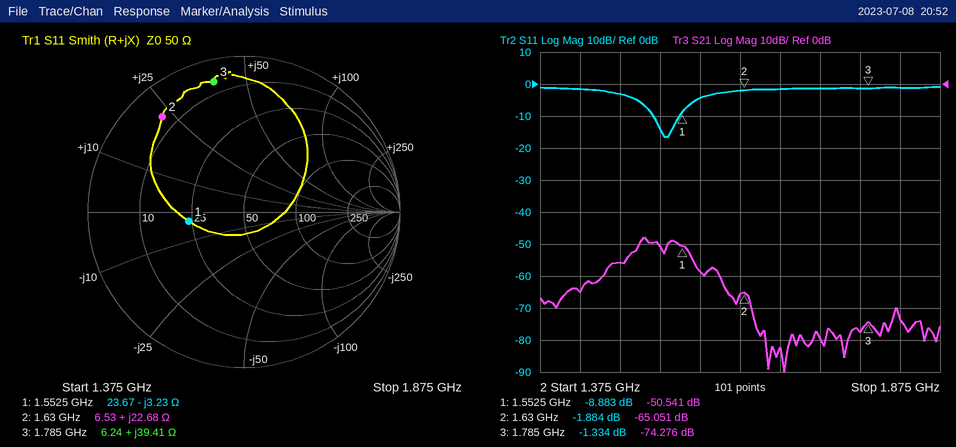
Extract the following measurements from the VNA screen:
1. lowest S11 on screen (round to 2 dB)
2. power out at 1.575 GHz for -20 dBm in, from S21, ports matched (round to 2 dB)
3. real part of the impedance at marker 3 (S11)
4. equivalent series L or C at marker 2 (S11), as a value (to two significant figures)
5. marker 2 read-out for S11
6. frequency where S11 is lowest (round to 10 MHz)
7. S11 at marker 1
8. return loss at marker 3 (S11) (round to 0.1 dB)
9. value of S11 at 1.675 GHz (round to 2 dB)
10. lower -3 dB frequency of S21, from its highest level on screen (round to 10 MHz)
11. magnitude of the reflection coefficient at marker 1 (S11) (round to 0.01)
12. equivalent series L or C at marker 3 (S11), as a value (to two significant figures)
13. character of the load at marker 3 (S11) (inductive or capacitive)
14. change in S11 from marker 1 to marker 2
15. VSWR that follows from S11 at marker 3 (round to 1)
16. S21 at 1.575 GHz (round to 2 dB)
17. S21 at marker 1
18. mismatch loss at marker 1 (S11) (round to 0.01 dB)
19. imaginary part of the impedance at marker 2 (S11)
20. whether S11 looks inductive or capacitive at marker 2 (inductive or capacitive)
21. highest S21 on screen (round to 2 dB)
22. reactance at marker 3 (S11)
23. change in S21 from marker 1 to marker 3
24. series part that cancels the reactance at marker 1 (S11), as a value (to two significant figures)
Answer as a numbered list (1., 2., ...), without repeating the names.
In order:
1. -16 dB
2. -78 dBm
3. 6.24 Ω
4. 2.2 nH
5. -1.884 dB
6. 1.53 GHz
7. -8.883 dB
8. 1.3 dB
9. -2 dB
10. 1.50 GHz
11. 0.36
12. 3.5 nH
13. inductive
14. 6.999 dB
15. 13
16. -58 dB
17. -50.541 dB
18. 0.60 dB
19. +22.68 Ω
20. inductive
21. -48 dB
22. +39.41 Ω
23. -23.735 dB
24. 330 pH
